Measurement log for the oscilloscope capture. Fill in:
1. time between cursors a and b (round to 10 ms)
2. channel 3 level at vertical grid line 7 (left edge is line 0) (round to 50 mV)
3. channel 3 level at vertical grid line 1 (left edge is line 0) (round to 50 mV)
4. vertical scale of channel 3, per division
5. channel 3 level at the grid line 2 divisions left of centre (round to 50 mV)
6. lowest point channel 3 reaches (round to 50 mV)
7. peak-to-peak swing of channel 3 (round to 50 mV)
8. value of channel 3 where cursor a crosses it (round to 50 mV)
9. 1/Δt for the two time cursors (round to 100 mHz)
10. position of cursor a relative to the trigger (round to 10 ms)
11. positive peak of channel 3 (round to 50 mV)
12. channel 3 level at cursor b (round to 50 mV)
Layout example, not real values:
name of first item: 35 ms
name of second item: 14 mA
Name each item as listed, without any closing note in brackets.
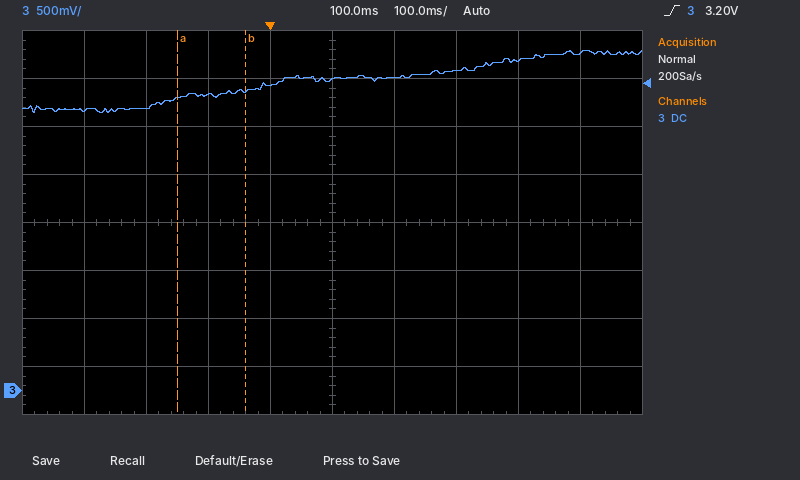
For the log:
time between cursors a and b: 110 ms
channel 3 level at vertical grid line 7 (left edge is line 0): 3.35 V
channel 3 level at vertical grid line 1 (left edge is line 0): 2.90 V
vertical scale of channel 3, per division: 500 mV
channel 3 level at the grid line 2 divisions left of centre: 3.10 V
lowest point channel 3 reaches: 2.90 V
peak-to-peak swing of channel 3: 650 mV
value of channel 3 where cursor a crosses it: 3.05 V
1/Δt for the two time cursors: 9.1 Hz
position of cursor a relative to the trigger: -150 ms
positive peak of channel 3: 3.55 V
channel 3 level at cursor b: 3.10 V
